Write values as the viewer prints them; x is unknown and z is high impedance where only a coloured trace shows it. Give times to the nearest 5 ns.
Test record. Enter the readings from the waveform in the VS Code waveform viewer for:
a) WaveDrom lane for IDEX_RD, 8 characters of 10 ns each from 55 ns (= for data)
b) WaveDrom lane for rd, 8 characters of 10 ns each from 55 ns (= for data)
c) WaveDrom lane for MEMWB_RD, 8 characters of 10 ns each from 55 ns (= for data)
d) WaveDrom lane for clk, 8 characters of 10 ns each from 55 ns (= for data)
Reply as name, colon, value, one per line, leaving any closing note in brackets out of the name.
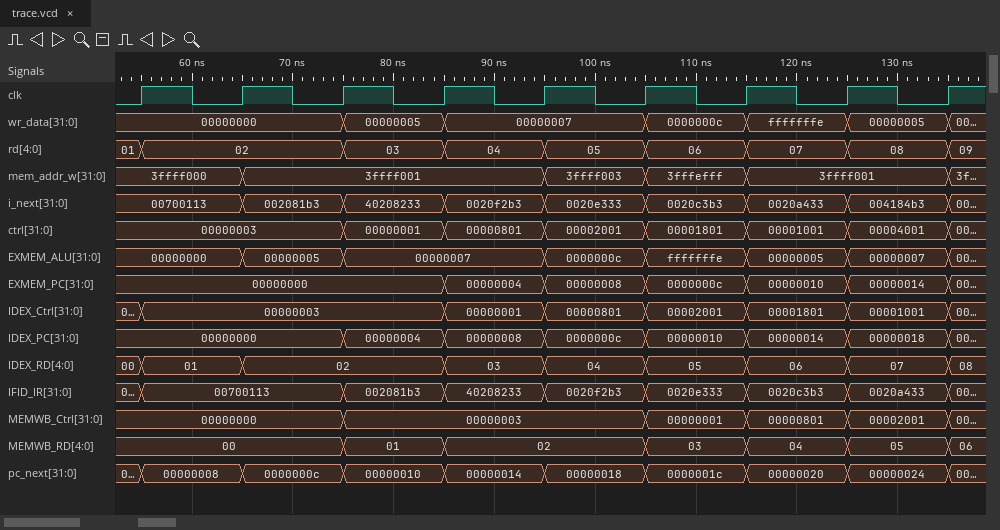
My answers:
WaveDrom lane for IDEX_RD, 8 characters of 10 ns each from 55 ns: {name: 'IDEX_RD', wave: '==.=====', data: '01 02 03 04 05 06 07'}
WaveDrom lane for rd, 8 characters of 10 ns each from 55 ns: {name: 'rd', wave: '=.======', data: '02 03 04 05 06 07 08'}
WaveDrom lane for MEMWB_RD, 8 characters of 10 ns each from 55 ns: {name: 'MEMWB_RD', wave: '=.==.===', data: '00 01 02 03 04 05'}
WaveDrom lane for clk, 8 characters of 10 ns each from 55 ns: {name: 'clk', wave: 'p.......'}
